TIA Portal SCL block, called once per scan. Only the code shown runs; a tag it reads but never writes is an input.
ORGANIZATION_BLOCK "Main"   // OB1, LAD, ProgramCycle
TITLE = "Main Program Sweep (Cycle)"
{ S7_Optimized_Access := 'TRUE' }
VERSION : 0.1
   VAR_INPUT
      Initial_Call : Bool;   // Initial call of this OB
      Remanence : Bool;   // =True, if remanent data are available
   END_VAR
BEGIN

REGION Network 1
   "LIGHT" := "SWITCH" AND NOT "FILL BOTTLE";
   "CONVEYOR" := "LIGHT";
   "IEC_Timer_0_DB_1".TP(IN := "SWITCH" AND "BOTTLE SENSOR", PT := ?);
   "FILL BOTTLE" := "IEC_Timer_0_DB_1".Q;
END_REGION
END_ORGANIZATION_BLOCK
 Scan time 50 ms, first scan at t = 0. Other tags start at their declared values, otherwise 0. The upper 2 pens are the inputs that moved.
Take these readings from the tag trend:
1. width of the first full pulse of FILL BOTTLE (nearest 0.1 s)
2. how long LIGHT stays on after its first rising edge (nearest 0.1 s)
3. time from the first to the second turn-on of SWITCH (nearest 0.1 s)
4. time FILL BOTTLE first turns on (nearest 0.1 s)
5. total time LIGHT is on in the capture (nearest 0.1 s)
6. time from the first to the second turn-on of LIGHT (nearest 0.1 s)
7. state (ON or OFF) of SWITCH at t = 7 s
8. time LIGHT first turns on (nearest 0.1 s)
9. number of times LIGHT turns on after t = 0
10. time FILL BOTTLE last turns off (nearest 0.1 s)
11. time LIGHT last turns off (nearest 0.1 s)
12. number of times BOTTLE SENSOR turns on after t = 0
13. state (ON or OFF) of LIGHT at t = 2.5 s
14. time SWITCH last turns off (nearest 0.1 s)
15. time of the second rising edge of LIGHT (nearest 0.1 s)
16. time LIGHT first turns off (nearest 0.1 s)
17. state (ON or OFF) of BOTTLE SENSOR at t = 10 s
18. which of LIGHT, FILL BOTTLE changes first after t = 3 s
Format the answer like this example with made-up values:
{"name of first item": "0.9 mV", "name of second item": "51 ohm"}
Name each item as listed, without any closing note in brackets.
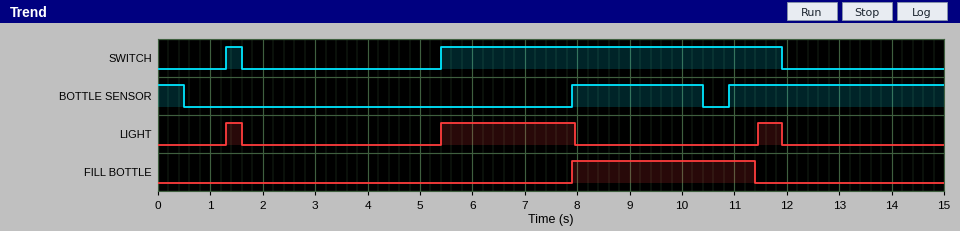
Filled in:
{"width of the first full pulse of FILL BOTTLE": "3.5 s", "how long LIGHT stays on after its first rising edge": "0.3 s", "time from the first to the second turn-on of SWITCH": "4.1 s", "time FILL BOTTLE first turns on": "7.9 s", "total time LIGHT is on in the capture": "3.3 s", "time from the first to the second turn-on of LIGHT": "4.1 s", "state (ON or OFF) of SWITCH at t = 7 s": "ON", "time LIGHT first turns on": "1.3 s", "number of times LIGHT turns on after t = 0": "3", "time FILL BOTTLE last turns off": "11.4 s", "time LIGHT last turns off": "11.9 s", "number of times BOTTLE SENSOR turns on after t = 0": "2", "state (ON or OFF) of LIGHT at t = 2.5 s": "OFF", "time SWITCH last turns off": "11.9 s", "time of the second rising edge of LIGHT": "5.4 s", "time LIGHT first turns off": "1.6 s", "state (ON or OFF) of BOTTLE SENSOR at t = 10 s": "ON", "which of LIGHT, FILL BOTTLE changes first after t = 3 s": "LIGHT"}
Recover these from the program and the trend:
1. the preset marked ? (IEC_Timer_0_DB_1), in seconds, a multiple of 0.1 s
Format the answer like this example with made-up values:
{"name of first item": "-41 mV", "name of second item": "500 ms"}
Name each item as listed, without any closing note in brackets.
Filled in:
{"the preset marked ? (IEC_Timer_0_DB_1), in seconds, a multiple of 0.1 s": "3.5 s"}
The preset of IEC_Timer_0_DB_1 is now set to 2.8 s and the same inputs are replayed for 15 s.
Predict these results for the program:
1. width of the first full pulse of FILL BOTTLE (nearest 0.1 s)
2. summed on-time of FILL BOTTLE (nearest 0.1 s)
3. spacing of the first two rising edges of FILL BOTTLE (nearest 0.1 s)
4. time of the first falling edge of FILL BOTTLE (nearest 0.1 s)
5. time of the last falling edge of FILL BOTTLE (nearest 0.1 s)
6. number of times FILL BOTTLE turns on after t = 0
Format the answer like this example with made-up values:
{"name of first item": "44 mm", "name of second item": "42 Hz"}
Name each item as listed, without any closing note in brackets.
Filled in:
{"width of the first full pulse of FILL BOTTLE": "2.8 s", "summed on-time of FILL BOTTLE": "5.6 s", "spacing of the first two rising edges of FILL BOTTLE": "3.0 s", "time of the first falling edge of FILL BOTTLE": "10.7 s", "time of the last falling edge of FILL BOTTLE": "13.7 s", "number of times FILL BOTTLE turns on after t = 0": "2"}
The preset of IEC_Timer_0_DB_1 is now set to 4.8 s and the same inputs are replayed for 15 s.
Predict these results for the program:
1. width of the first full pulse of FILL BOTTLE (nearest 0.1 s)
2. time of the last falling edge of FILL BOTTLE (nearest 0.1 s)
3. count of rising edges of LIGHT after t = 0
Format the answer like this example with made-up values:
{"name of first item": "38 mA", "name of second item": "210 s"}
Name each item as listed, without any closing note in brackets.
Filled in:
{"width of the first full pulse of FILL BOTTLE": "4.8 s", "time of the last falling edge of FILL BOTTLE": "12.7 s", "count of rising edges of LIGHT after t = 0": "2"}
